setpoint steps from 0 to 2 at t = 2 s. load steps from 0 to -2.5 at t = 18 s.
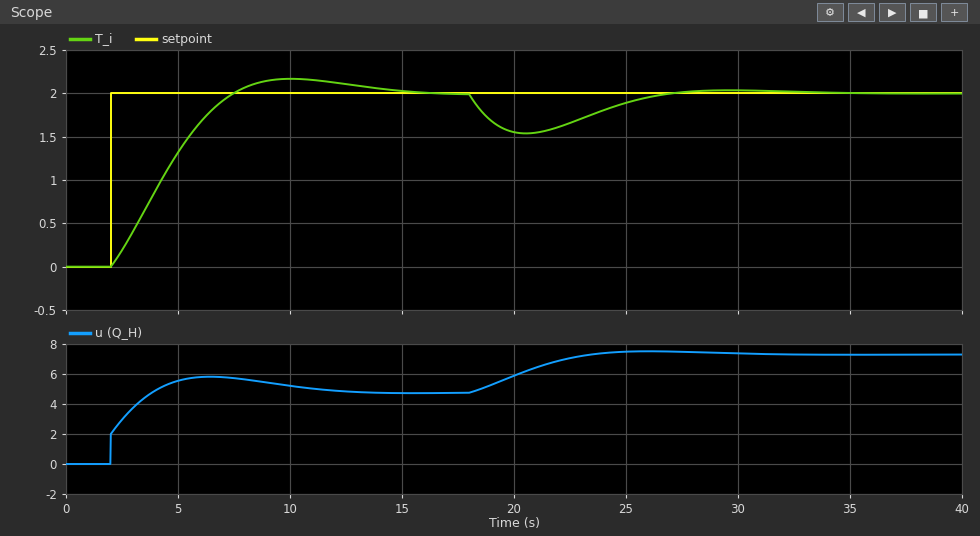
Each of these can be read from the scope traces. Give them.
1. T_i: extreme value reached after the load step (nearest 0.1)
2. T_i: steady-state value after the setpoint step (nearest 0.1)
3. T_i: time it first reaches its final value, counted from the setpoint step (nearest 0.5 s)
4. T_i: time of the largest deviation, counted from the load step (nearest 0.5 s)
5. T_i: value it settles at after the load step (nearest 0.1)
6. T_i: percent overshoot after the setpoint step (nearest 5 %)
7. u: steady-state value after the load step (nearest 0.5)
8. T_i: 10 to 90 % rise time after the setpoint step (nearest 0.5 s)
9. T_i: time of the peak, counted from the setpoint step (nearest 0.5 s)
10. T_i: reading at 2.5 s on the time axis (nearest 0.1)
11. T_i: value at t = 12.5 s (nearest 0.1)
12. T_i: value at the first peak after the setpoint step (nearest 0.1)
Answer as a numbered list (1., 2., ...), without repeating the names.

1. 1.5
2. 2.0
3. 5.5 s
4. 2.5 s
5. 2.0
6. 10 %
7. 7.5
8. 4.0 s
9. 8.0 s
10. 0.2
11. 2.1
12. 2.2
